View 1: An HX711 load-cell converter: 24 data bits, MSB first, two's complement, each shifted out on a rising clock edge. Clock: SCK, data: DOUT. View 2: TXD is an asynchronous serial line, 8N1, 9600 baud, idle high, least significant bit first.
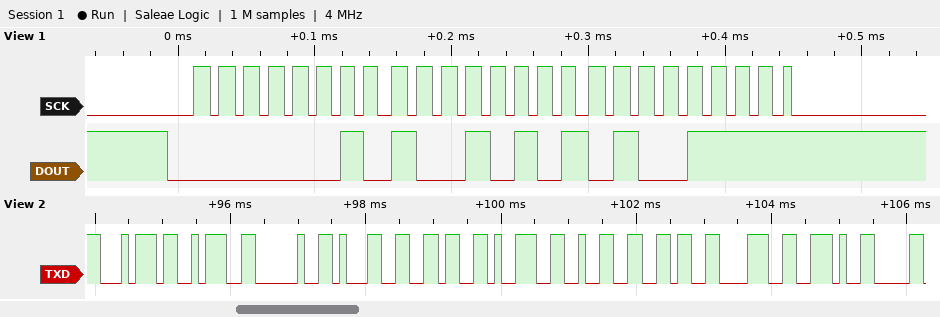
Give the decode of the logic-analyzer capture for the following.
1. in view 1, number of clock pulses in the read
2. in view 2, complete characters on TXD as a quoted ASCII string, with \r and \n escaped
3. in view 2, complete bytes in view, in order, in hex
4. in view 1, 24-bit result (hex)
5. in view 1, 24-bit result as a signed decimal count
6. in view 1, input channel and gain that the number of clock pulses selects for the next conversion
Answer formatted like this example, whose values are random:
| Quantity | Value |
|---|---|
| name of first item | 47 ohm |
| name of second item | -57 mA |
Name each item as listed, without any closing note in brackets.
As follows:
| Quantity | Value |
|---|---|
| in view 1, number of clock pulses in the read | 25 |
| in view 2, complete characters on TXD as a quoted ASCII string, with \r and \n escaped | "t: 169268." |
| in view 2, complete bytes in view, in order, in hex | 74 3A 20 31 36 39 32 36 38 2E |
| in view 1, 24-bit result | 0x02954F |
| in view 1, 24-bit result as a signed decimal count | 169295 |
| in view 1, input channel and gain that the number of clock pulses selects for the next conversion | channel A, gain 128 |
